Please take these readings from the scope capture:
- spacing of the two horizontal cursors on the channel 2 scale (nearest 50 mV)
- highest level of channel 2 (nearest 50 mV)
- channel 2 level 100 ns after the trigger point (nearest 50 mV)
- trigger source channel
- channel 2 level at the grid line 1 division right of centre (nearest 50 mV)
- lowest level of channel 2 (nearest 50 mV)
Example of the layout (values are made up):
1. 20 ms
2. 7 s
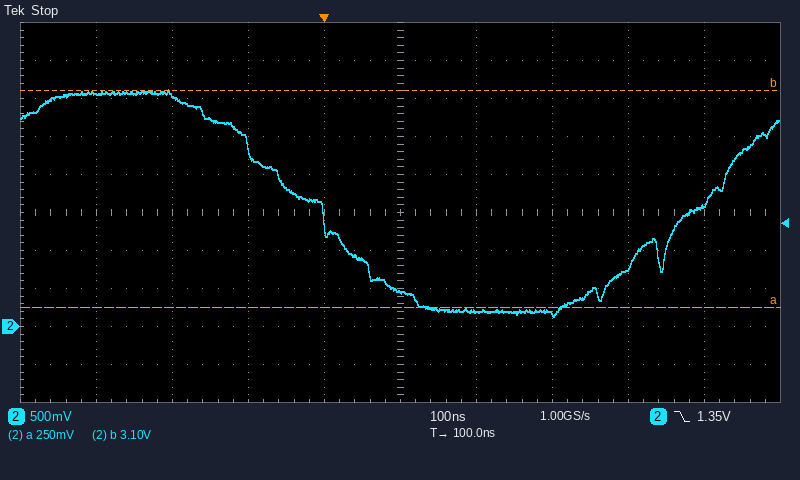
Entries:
1. 2.85 V
2. 3.10 V
3. 450 mV
4. channel 2
5. 200 mV
6. 150 mV
